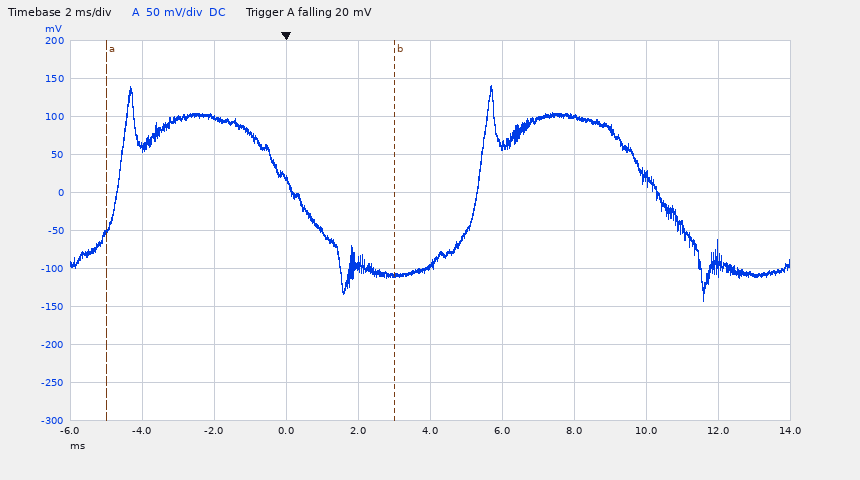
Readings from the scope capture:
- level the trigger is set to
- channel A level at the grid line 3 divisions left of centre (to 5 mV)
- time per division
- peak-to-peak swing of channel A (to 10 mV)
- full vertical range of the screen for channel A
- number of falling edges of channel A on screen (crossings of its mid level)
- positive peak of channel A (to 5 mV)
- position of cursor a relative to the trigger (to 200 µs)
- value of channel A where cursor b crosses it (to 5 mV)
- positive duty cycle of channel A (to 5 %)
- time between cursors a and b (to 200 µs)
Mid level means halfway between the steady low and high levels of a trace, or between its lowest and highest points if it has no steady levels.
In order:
20 mV
100 mV
2 ms
280 mV
500 mV
2
140 mV
-5.0 ms
-110 mV
50 %
8.0 ms
